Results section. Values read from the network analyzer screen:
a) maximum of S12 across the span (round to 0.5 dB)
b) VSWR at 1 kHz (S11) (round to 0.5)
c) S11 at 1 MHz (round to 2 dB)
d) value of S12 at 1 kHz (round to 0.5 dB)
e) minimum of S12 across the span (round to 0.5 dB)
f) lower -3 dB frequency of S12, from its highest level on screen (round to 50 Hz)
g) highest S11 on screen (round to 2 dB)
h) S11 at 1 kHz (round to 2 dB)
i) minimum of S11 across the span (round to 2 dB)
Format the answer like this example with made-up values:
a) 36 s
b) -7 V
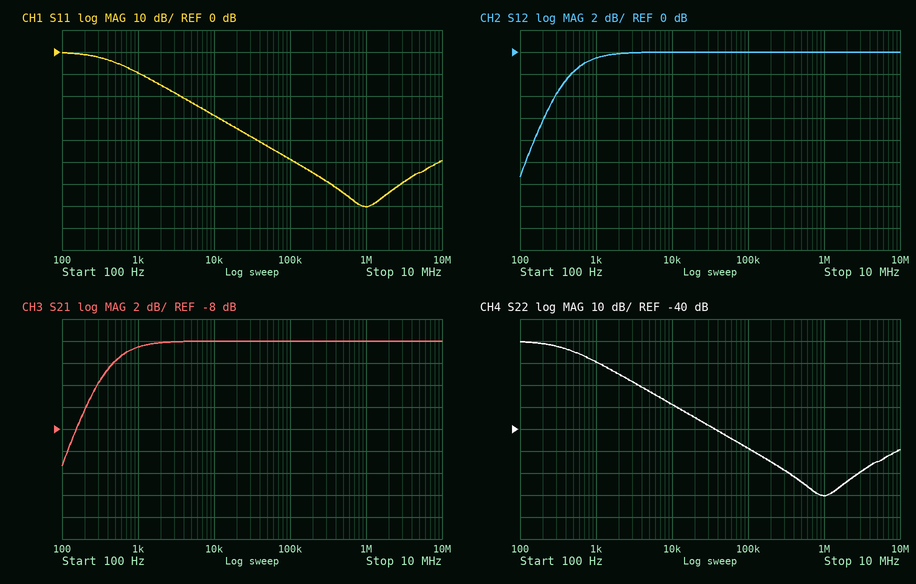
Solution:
a) 0.0 dB
b) 2.0
c) -70 dB
d) -0.5 dB
e) -11.5 dB
f) 350 Hz
g) 0 dB
h) -10 dB
i) -70 dB
